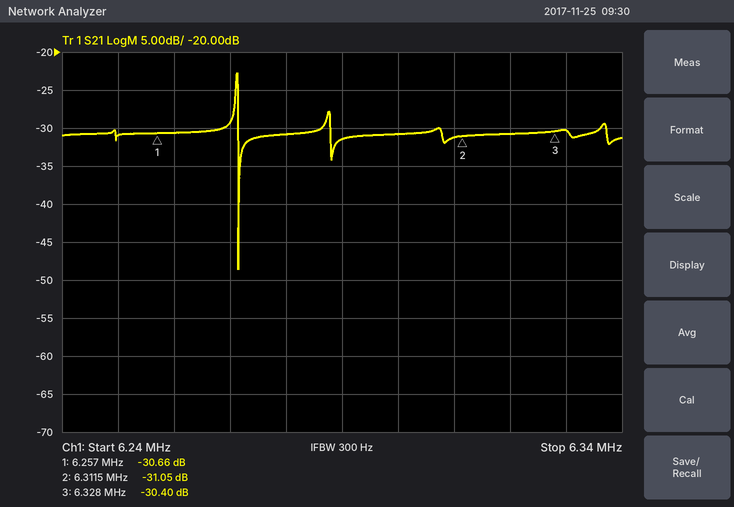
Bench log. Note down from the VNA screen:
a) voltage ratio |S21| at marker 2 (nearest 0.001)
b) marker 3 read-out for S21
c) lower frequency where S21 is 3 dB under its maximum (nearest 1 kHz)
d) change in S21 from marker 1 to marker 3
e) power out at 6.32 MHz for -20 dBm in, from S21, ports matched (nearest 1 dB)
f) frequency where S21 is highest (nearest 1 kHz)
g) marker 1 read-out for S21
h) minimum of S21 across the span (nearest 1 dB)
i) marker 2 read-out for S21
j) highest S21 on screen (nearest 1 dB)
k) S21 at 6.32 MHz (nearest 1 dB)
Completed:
0.028
-30.40 dB
6.271 MHz
0.26 dB
-51 dBm
6.271 MHz
-30.66 dB
-49 dB
-31.05 dB
-23 dB
-31 dB
